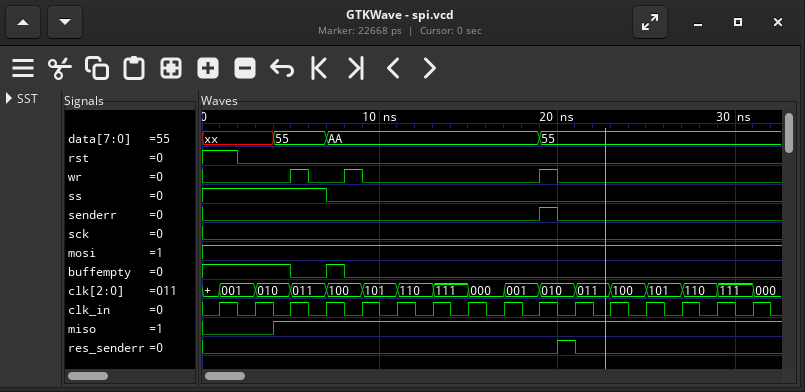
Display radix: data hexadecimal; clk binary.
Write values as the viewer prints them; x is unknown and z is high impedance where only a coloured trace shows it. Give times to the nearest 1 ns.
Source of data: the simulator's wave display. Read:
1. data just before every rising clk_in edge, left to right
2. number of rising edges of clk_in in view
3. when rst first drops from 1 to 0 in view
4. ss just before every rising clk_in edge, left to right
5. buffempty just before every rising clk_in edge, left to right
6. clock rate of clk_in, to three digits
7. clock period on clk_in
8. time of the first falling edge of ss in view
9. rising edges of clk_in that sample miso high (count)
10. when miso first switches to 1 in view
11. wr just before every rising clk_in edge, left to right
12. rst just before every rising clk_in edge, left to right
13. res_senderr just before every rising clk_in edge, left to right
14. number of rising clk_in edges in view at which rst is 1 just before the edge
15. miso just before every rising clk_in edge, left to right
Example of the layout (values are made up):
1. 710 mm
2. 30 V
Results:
1. xx, xx, 55, 55, AA, AA, AA, AA, AA, AA, 55, 55, 55, 55, 55, 55
2. 16
3. 2 ns
4. 1 1 1 1 0 0 0 0 0 0 0 0 0 0 0 0
5. 1 1 1 0 0 0 0 0 0 0 0 0 0 0 0 0
6. 500 MHz
7. 2 ns
8. 7 ns
9. 14
10. 4 ns
11. 0 0 0 0 1 0 0 0 0 0 0 0 0 0 0 0
12. 1 0 0 0 0 0 0 0 0 0 0 0 0 0 0 0
13. 0 0 0 0 0 0 0 0 0 0 1 0 0 0 0 0
14. 1
15. 0 0 1 1 1 1 1 1 1 1 1 1 1 1 1 1
